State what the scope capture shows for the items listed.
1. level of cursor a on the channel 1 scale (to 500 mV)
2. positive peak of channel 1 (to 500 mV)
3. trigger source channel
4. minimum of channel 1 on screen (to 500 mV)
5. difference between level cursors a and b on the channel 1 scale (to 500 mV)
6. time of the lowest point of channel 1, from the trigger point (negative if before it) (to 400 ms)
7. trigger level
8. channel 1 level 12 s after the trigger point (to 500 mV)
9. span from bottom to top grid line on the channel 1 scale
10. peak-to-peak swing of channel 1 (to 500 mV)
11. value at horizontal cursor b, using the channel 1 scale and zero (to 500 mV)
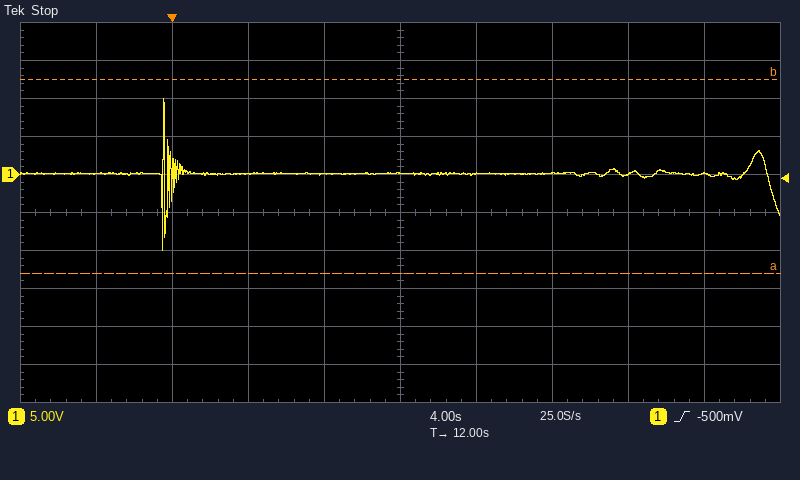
-13.0 V
10.0 V
channel 1
-10.0 V
25.5 V
-400 ms
-500 mV
0.0 V
50 V
20.0 V
12.5 V
